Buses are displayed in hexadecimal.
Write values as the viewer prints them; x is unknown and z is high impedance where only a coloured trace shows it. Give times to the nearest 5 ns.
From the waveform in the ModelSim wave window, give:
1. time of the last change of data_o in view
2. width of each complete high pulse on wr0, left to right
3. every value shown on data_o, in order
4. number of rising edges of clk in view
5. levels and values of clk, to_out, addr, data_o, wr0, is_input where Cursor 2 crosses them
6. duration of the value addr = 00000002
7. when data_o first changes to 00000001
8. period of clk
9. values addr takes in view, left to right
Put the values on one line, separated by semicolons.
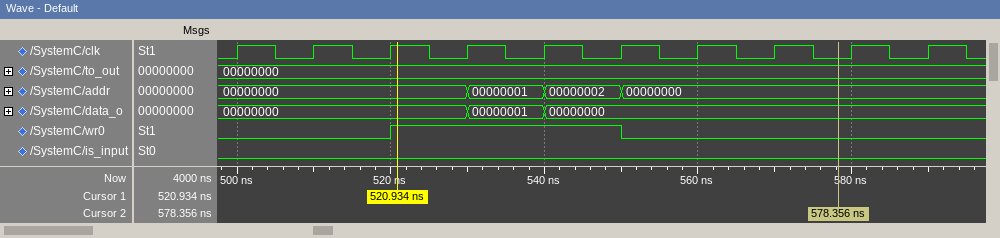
540 ns; 30 ns; 00000000, 00000001, 00000000; 10; clk=0, to_out=00000000, addr=00000000, data_o=00000000, wr0=0, is_input=0; 10 ns; 530 ns; 10 ns; 00000000, 00000001, 00000002, 00000000
